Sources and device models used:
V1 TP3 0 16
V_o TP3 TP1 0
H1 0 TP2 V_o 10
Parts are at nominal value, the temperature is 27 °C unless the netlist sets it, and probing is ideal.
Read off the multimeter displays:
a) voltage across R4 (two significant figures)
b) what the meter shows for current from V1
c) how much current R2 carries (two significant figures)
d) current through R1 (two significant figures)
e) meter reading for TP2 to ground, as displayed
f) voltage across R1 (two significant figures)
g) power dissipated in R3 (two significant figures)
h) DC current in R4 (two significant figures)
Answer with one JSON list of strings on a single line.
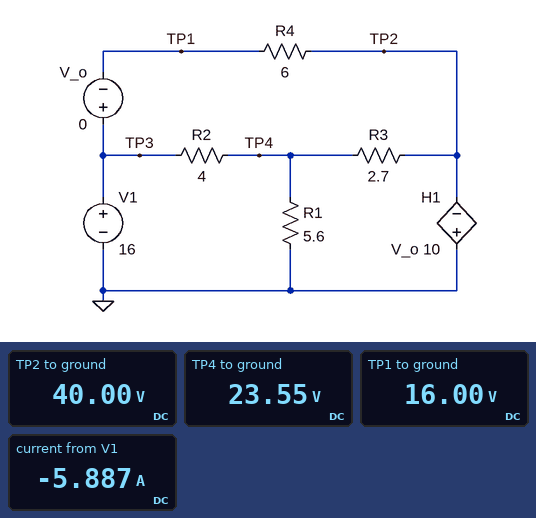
["24 V", "-5.887 A", "1.9 A", "4.2 A", "40.00 V", "24 V", "100 W", "4.0 A"]
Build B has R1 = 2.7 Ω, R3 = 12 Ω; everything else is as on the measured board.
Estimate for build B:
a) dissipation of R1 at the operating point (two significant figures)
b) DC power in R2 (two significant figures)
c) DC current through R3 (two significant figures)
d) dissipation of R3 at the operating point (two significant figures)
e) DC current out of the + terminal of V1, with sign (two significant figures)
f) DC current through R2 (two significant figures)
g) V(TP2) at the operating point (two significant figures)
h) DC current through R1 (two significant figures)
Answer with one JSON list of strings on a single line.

["40 W", "7.8 W", "2.5 A", "73 W", "-2.6 A", "1.4 A", "40 V", "3.9 A"]
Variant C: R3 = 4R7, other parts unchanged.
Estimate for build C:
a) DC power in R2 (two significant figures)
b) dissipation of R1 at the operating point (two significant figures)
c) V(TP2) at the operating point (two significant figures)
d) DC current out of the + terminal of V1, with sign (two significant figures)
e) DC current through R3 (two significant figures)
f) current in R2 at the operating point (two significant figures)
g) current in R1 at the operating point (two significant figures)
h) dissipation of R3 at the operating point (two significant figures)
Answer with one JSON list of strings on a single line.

["3.1 W", "68 W", "40 V", "-4.9 A", "4.4 A", "880 mA", "3.5 A", "89 W"]
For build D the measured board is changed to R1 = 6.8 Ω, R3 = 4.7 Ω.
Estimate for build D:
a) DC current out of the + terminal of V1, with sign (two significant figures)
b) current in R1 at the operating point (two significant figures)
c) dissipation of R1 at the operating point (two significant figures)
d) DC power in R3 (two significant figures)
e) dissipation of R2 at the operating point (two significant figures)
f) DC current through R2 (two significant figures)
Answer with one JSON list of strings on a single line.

["-5.1 A", "3.0 A", "62 W", "81 W", "5.1 W", "1.1 A"]
